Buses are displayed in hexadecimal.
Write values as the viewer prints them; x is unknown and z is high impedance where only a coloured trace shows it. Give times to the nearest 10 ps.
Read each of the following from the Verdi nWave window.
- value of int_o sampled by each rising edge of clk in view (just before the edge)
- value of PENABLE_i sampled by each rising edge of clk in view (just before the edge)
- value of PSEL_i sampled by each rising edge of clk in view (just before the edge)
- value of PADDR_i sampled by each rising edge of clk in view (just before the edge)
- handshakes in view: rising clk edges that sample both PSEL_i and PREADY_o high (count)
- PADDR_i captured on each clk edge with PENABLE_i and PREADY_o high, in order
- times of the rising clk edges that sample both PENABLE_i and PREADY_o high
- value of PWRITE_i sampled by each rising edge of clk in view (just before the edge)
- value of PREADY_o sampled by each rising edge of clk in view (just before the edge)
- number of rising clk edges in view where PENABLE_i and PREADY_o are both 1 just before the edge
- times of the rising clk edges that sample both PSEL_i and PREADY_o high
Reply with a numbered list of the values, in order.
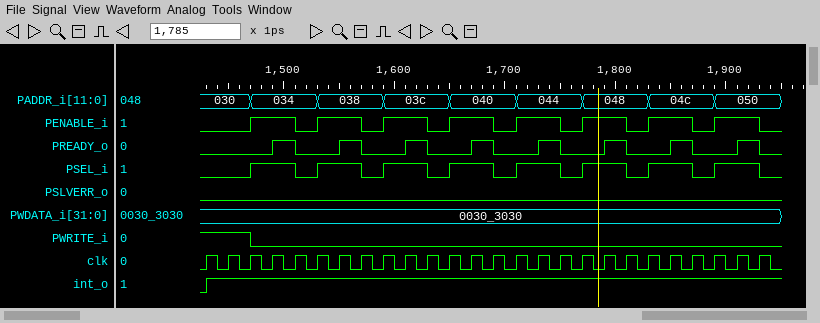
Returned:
1. 0 1 1 1 1 1 1 1 1 1 1 1 1 1 1 1 1 1 1 1 1 1 1 1 1 1
2. 0 0 0 1 1 0 1 1 0 1 1 0 1 1 0 1 1 0 1 1 0 1 1 0 1 1
3. 0 0 0 1 1 0 1 1 0 1 1 0 1 1 0 1 1 0 1 1 0 1 1 0 1 1
4. 030, 030, 030, 034, 034, 034, 038, 038, 038, 03c, 03c, 03c, 040, 040, 040, 044, 044, 044, 048, 048, 048, 04c, 04c, 04c, 050, 050
5. 8
6. 034, 038, 03c, 040, 044, 048, 04c, 050
7. 1510 ps, 1570 ps, 1630 ps, 1690 ps, 1750 ps, 1810 ps, 1870 ps, 1930 ps
8. 1 1 1 0 0 0 0 0 0 0 0 0 0 0 0 0 0 0 0 0 0 0 0 0 0 0
9. 0 0 0 0 1 0 0 1 0 0 1 0 0 1 0 0 1 0 0 1 0 0 1 0 0 1
10. 8
11. 1510 ps, 1570 ps, 1630 ps, 1690 ps, 1750 ps, 1810 ps, 1870 ps, 1930 ps
